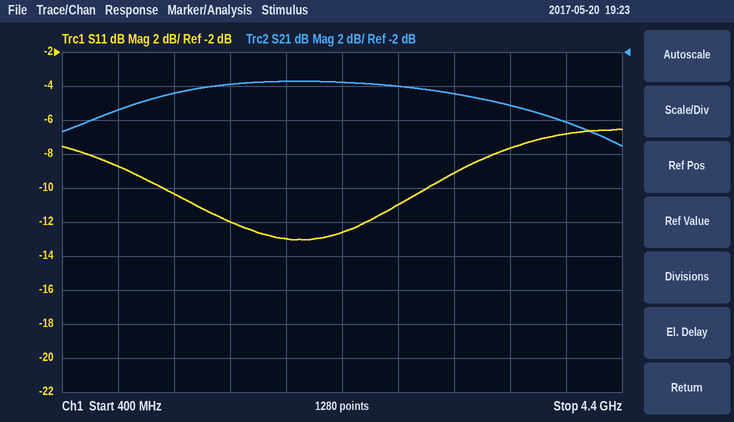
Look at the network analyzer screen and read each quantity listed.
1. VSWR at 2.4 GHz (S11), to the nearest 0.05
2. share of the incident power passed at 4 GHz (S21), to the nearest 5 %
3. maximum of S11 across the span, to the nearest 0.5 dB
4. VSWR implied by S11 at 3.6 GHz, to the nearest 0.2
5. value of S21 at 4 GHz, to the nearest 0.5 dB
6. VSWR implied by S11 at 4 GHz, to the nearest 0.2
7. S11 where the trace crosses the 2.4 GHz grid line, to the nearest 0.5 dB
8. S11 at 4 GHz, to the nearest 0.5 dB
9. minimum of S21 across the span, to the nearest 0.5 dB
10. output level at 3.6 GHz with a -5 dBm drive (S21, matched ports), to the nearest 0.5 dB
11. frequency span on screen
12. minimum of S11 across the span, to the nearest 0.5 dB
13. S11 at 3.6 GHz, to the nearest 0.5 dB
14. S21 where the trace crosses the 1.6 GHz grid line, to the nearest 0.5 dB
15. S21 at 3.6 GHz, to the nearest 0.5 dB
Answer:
1.60
25 %
-6.5 dB
2.4
-6.0 dB
2.6
-12.5 dB
-7.0 dB
-7.5 dB
-10.0 dBm
4 GHz
-13.0 dB
-7.5 dB
-4.0 dB
-5.0 dB
